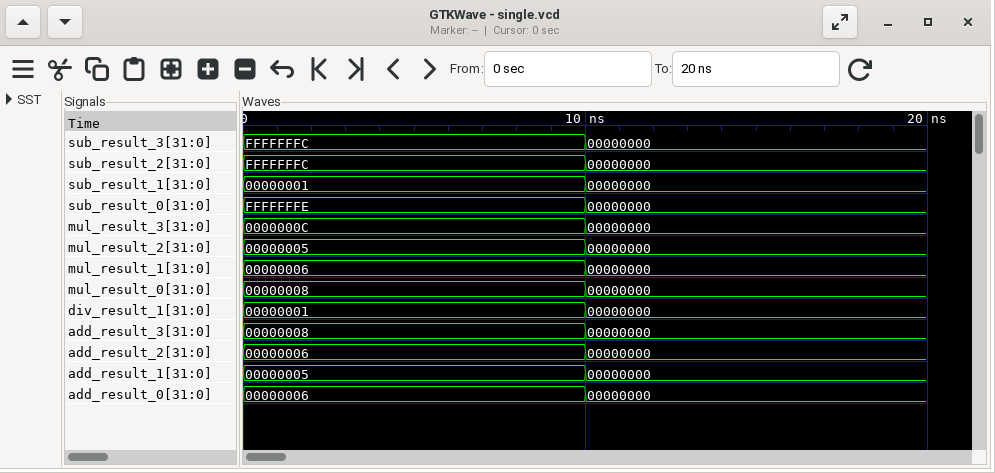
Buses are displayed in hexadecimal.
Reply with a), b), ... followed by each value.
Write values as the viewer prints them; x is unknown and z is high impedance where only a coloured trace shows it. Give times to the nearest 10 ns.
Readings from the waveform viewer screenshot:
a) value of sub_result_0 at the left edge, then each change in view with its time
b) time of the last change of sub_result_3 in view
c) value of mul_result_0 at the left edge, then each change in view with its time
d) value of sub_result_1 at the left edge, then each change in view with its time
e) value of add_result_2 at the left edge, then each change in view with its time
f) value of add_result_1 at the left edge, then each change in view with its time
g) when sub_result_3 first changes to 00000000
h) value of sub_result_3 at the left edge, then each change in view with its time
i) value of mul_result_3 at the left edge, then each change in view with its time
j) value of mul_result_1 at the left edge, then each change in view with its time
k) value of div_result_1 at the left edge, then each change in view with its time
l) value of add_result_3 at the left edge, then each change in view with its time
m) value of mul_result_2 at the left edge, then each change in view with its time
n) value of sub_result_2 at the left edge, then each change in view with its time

a) FFFFFFFE, 00000000 at 10 ns
b) 10 ns
c) 00000008, 00000000 at 10 ns
d) 00000001, 00000000 at 10 ns
e) 00000006, 00000000 at 10 ns
f) 00000005, 00000000 at 10 ns
g) 10 ns
h) FFFFFFFC, 00000000 at 10 ns
i) 0000000C, 00000000 at 10 ns
j) 00000006, 00000000 at 10 ns
k) 00000001, 00000000 at 10 ns
l) 00000008, 00000000 at 10 ns
m) 00000005, 00000000 at 10 ns
n) FFFFFFFC, 00000000 at 10 ns
